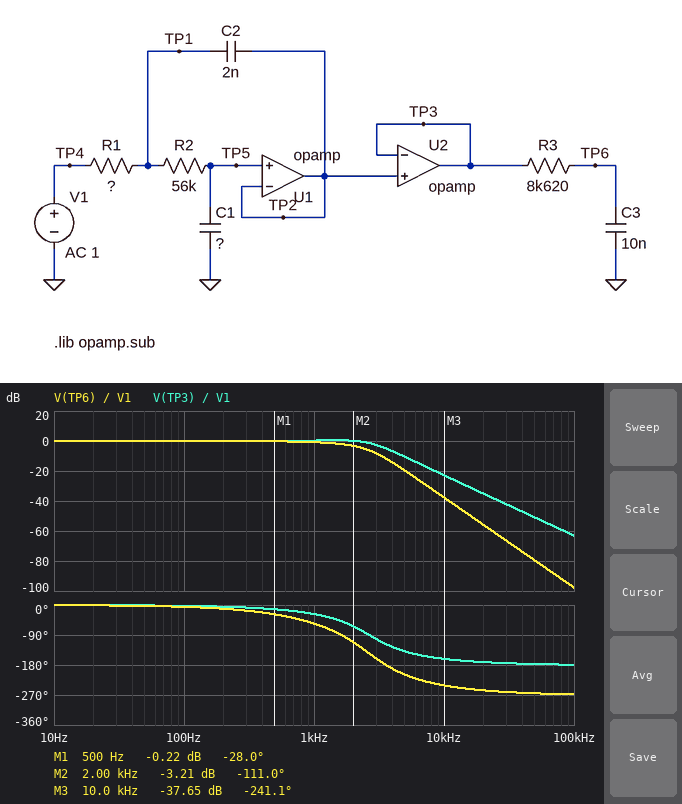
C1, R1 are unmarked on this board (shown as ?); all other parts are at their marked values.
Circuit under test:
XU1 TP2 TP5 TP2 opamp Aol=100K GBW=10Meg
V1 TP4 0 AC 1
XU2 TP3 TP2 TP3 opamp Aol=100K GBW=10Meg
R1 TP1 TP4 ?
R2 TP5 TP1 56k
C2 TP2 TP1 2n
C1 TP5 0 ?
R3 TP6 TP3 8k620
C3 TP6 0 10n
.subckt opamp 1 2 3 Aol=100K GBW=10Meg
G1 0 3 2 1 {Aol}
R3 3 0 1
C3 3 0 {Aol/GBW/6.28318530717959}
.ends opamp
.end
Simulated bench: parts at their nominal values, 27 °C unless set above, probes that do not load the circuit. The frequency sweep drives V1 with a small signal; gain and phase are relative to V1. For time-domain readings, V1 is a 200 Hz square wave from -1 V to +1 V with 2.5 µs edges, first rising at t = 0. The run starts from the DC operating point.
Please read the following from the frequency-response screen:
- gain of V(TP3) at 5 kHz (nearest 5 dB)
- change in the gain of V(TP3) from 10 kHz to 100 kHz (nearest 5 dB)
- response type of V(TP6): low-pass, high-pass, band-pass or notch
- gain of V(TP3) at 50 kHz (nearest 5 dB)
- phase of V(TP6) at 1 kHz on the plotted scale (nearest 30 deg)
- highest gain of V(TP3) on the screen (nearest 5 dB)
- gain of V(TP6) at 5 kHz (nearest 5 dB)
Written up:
-10 dB
-40 dB
low-pass
-50 dB
-60 deg
0 dB
-20 dB
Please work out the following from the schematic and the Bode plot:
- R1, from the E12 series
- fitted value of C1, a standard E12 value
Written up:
47 kΩ
680 pF
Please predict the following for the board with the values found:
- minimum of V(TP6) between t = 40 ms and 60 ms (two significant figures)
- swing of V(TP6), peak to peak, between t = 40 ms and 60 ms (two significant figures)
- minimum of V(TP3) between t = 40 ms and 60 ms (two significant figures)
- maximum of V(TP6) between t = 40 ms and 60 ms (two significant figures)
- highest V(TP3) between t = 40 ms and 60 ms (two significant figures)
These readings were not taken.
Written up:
-1.0 V
2.0 V
-1.2 V
1.0 V
1.2 V
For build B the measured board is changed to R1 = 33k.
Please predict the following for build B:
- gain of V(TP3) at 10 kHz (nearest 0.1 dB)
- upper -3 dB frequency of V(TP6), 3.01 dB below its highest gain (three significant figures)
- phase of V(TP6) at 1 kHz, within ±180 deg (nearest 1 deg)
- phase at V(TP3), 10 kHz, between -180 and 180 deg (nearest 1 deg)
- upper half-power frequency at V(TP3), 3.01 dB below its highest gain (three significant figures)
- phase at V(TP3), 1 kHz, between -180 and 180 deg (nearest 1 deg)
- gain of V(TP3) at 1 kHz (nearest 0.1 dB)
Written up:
-19.7 dB
1.96 kHz
-51 deg
-157 deg
3.53 kHz
-23 deg
0.2 dB
